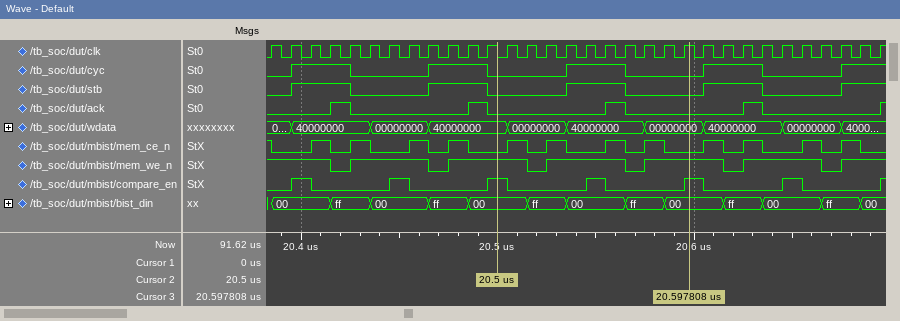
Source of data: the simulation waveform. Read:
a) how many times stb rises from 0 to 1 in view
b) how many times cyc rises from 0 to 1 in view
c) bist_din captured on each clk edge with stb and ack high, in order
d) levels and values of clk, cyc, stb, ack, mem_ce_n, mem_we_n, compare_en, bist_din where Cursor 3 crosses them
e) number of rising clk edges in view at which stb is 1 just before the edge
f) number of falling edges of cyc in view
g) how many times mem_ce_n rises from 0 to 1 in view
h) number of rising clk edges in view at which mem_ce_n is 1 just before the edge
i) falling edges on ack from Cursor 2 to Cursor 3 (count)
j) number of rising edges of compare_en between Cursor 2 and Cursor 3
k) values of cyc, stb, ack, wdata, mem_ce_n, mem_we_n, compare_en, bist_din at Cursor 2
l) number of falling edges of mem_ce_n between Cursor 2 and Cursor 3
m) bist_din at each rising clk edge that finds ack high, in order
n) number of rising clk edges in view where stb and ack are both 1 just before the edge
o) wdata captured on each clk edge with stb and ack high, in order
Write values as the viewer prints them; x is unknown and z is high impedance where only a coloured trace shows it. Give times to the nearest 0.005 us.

5
5
ff, 00, 00, ff
clk=1, cyc=0, stb=0, ack=0, mem_ce_n=0, mem_we_n=1, compare_en=1, bist_din=00
14
4
12
13
1
2
cyc=0, stb=0, ack=0, wdata=40000000, mem_ce_n=0, mem_we_n=1, compare_en=1, bist_din=00
4
ff, 00, 00, ff
4
40000000, 40000000, 40000000, 40000000
